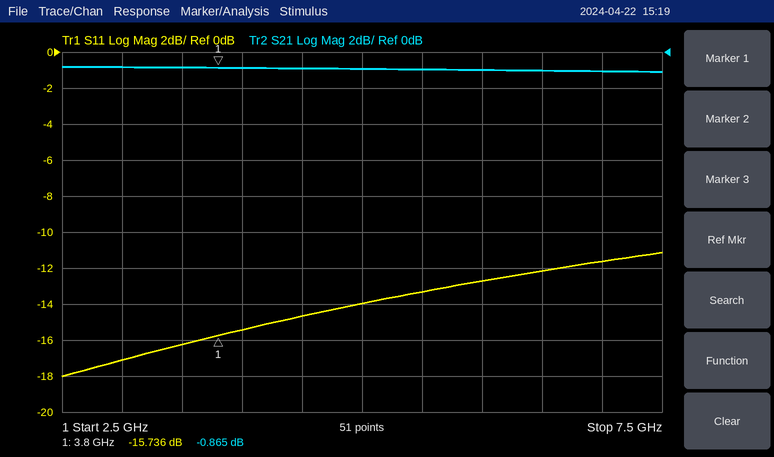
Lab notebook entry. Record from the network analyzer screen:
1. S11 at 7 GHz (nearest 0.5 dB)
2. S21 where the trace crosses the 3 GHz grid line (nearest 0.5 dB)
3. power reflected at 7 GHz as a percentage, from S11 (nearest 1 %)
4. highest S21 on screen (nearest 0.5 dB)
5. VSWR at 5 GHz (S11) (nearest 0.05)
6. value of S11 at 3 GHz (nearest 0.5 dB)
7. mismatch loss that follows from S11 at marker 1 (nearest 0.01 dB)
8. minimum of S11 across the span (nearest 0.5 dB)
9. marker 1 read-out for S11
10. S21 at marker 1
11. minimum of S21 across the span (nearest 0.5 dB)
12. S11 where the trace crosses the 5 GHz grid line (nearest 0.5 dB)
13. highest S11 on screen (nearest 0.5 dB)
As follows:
-11.5 dB
-1.0 dB
7 %
-1.0 dB
1.50
-17.0 dB
0.12 dB
-18.0 dB
-15.736 dB
-0.865 dB
-1.0 dB
-14.0 dB
-11.0 dB
